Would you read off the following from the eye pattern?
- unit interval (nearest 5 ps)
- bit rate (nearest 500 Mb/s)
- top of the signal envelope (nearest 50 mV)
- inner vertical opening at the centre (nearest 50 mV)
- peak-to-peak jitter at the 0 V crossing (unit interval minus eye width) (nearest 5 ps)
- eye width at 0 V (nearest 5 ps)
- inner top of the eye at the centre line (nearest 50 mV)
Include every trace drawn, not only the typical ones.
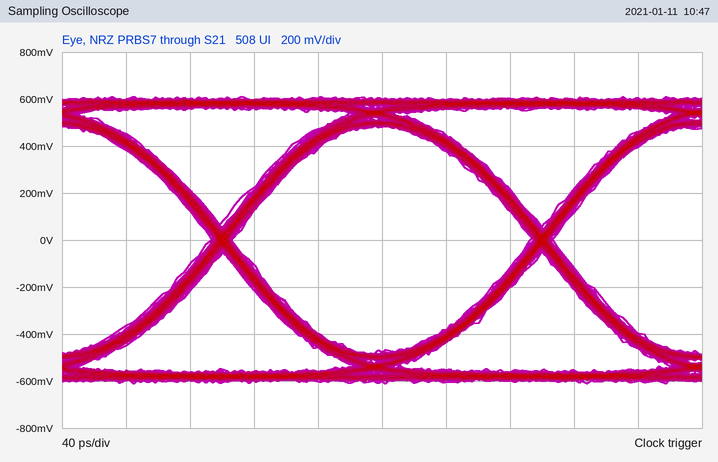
200 ps
5.0 Gb/s
600 mV
950 mV
15 ps
185 ps
500 mV
